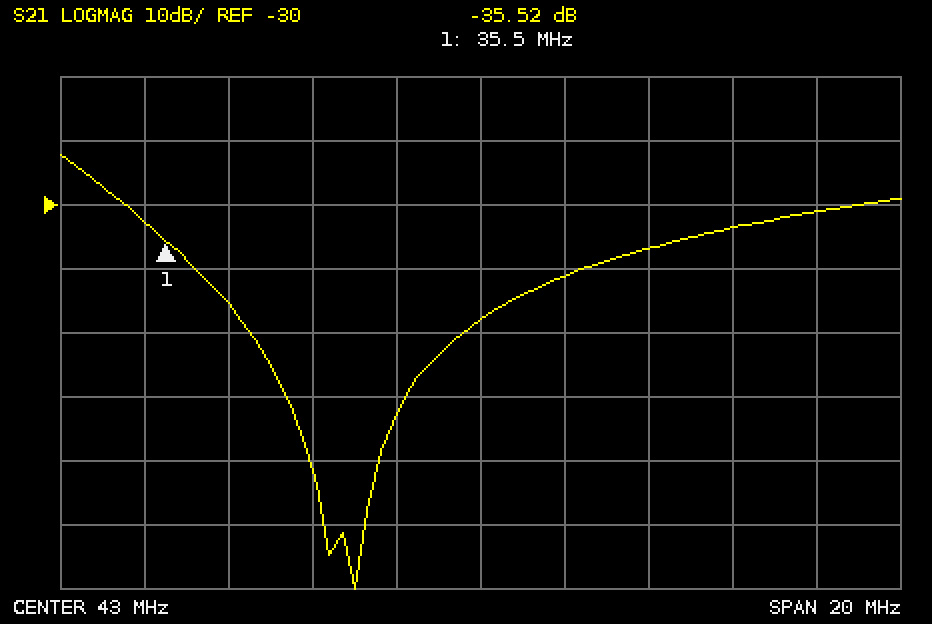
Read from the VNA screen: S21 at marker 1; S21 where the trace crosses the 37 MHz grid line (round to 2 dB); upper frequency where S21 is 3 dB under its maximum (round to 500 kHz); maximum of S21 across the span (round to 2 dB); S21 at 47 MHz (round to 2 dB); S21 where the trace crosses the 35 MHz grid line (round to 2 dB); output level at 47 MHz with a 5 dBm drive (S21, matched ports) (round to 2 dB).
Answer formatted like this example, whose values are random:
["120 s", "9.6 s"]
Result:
["-35.52 dB", "-46 dB", "33.5 MHz", "-22 dB", "-36 dB", "-32 dB", "-32 dBm"]
